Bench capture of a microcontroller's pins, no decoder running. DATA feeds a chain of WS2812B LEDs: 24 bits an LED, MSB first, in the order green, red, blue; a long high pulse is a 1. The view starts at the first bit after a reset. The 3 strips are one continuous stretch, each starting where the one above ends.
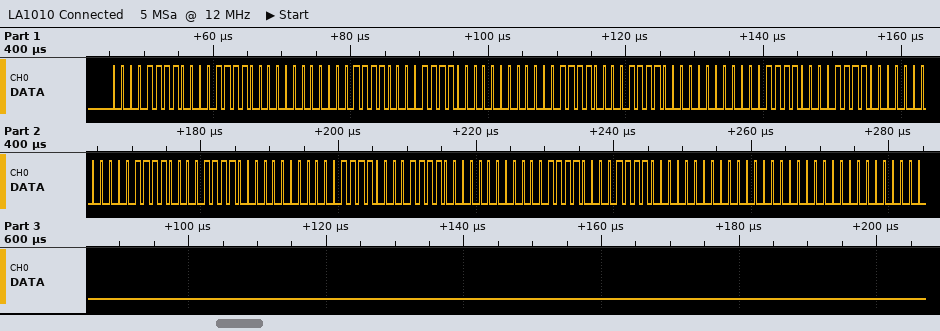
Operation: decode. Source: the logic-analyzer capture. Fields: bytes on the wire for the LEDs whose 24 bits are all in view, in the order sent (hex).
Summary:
0F 0F 00 0F 0F 00 0F 0F 00 0F 0F 00 0F 0F 00 0F 0F 00 0F 0F 00 00 00 00
